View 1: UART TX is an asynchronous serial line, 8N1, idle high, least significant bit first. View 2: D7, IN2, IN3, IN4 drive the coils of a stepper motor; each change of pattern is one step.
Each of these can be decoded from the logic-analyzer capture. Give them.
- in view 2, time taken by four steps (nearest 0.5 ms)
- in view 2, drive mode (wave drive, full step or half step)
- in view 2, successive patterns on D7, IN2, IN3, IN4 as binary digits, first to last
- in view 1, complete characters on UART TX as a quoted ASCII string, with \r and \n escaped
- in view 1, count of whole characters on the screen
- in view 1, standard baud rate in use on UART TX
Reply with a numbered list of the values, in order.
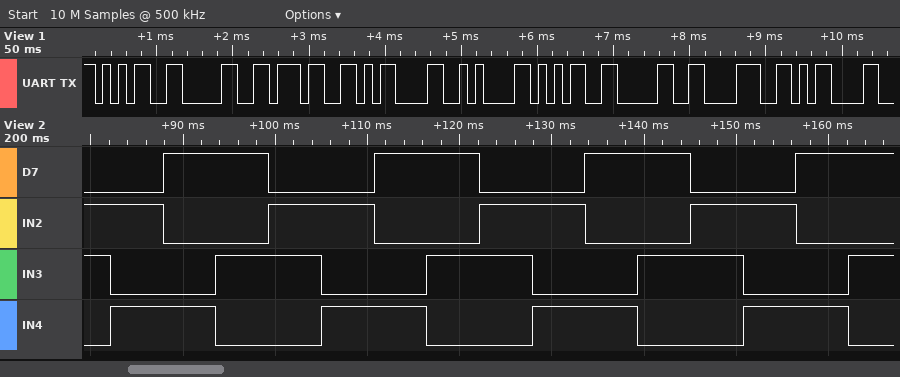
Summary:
1. 23.0 ms
2. full step
3. 0110 0101 1001 1010 0110 0101 1001 1010 0110 0101 1001 1010 0110 0101 1001 1010
4. "507\r\n508\r"
5. 9
6. 9600 baud
